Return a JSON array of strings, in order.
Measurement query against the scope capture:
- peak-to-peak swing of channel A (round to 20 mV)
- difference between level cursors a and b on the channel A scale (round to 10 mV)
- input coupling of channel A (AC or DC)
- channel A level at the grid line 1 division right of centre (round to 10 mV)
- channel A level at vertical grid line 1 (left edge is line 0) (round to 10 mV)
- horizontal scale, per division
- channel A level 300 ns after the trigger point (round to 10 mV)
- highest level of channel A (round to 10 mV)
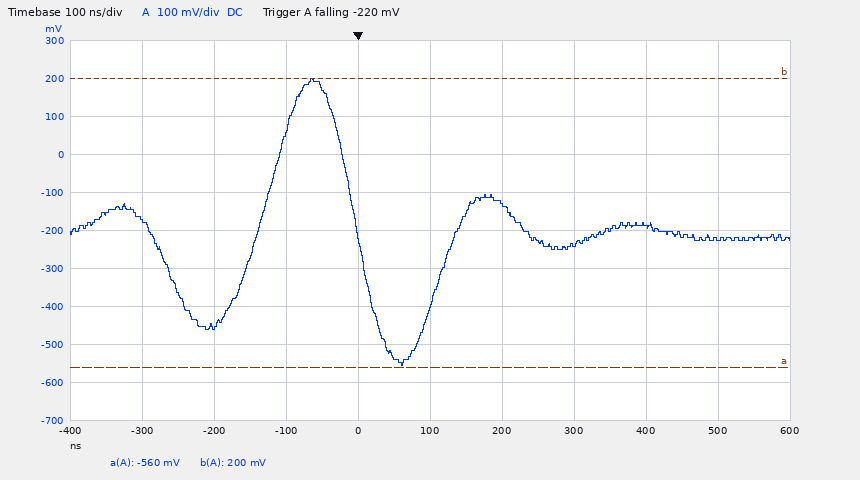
["760 mV", "760 mV", "DC", "-130 mV", "-170 mV", "100 ns", "-240 mV", "200 mV"]
